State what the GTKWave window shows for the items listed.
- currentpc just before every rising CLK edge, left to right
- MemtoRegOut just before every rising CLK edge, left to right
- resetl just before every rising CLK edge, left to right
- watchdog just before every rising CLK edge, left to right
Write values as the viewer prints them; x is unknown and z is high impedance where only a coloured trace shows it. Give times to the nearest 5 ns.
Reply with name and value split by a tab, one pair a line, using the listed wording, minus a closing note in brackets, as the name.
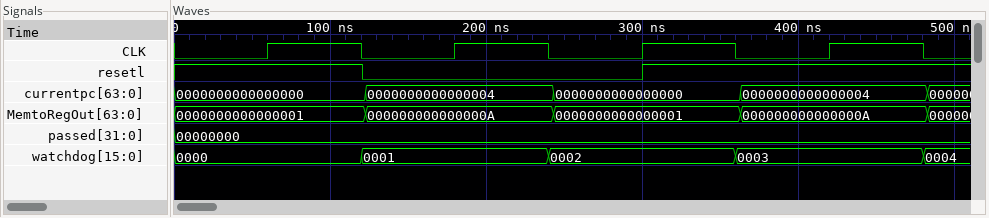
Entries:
currentpc just before every rising CLK edge, left to right	0000000000000000, 0000000000000004, 0000000000000000, 0000000000000004
MemtoRegOut just before every rising CLK edge, left to right	0000000000000001, 000000000000000A, 0000000000000001, 000000000000000A
resetl just before every rising CLK edge, left to right	1 0 0 1
watchdog just before every rising CLK edge, left to right	0000, 0001, 0002, 0003
